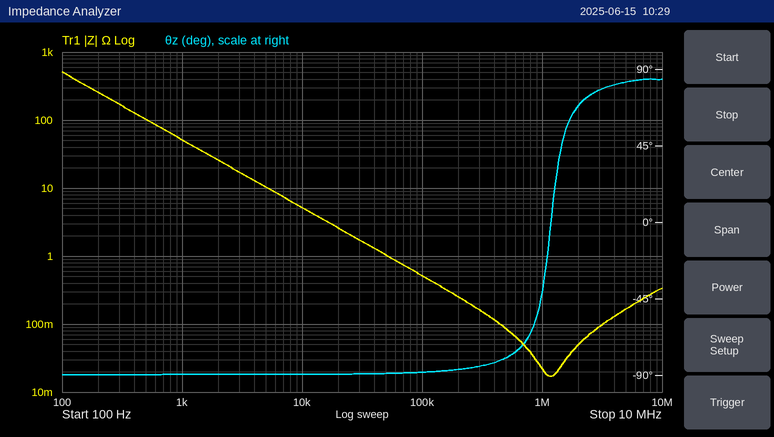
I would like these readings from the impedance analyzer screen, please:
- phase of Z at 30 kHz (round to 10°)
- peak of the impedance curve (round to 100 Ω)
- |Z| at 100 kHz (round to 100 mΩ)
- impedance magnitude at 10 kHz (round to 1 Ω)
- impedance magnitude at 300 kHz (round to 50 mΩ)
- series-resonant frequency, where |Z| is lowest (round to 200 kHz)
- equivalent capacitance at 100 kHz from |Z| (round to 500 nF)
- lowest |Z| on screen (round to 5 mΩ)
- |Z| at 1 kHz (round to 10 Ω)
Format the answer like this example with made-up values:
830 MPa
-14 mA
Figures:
-90°
500 Ω
500 mΩ
5 Ω
150 mΩ
1.2 MHz
3.0 µF
15 mΩ
50 Ω
